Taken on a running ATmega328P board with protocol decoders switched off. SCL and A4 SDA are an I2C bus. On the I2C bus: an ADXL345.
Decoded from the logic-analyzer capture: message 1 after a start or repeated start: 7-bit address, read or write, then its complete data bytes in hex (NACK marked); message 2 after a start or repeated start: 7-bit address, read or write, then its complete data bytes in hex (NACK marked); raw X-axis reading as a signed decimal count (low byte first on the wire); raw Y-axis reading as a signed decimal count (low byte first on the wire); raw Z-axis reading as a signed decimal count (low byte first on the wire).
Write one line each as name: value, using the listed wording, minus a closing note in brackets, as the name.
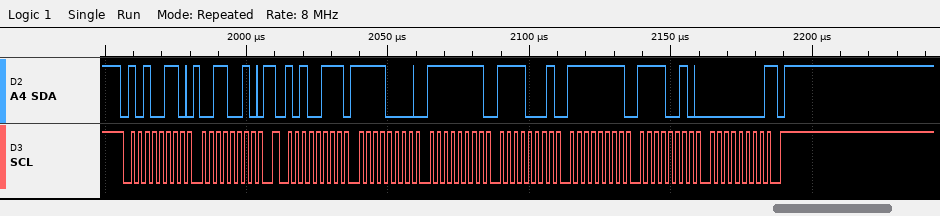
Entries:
message 1 after a start or repeated start: 7-bit address, read or write, then its complete data bytes in hex: 0x53 write: 32
message 2 after a start or repeated start: 7-bit address, read or write, then its complete data bytes in hex: 0x53 read: F0 FF F1 FF F2 00 NACK
raw X-axis reading as a signed decimal count: -16
raw Y-axis reading as a signed decimal count: -15
raw Z-axis reading as a signed decimal count: 242
